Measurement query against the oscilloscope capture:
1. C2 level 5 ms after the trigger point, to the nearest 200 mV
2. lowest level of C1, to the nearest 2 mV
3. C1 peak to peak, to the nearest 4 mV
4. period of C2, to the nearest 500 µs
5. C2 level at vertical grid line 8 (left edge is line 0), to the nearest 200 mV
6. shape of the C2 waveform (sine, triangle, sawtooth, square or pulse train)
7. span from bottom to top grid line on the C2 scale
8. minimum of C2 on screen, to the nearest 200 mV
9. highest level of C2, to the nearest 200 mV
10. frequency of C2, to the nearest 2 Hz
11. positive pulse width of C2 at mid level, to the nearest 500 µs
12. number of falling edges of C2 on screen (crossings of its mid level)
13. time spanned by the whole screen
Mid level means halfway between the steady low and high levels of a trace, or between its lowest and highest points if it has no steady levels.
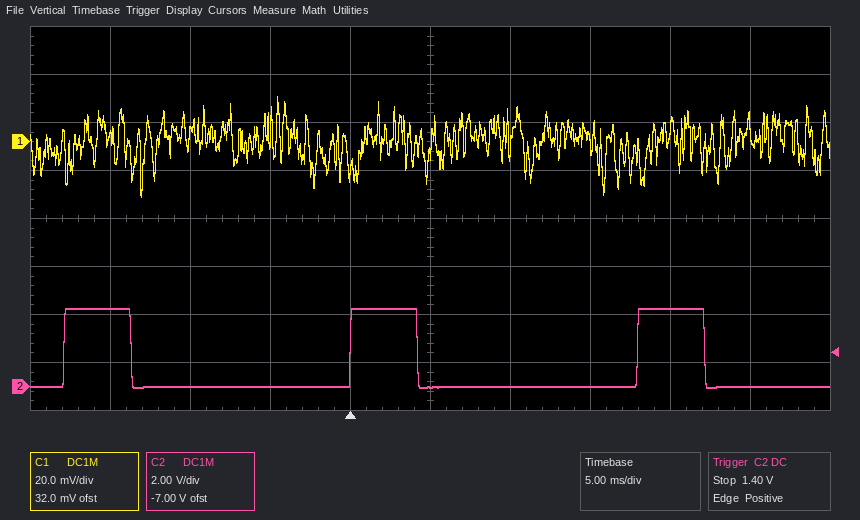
0.0 V
-22 mV
40 mV
18.0 ms
3.2 V
pulse train
16 V
0.0 V
3.2 V
56 Hz
4.0 ms
3
50 ms
